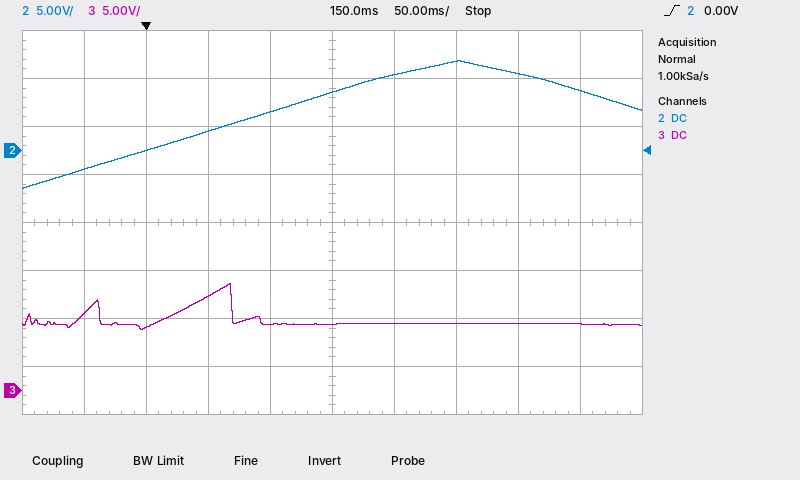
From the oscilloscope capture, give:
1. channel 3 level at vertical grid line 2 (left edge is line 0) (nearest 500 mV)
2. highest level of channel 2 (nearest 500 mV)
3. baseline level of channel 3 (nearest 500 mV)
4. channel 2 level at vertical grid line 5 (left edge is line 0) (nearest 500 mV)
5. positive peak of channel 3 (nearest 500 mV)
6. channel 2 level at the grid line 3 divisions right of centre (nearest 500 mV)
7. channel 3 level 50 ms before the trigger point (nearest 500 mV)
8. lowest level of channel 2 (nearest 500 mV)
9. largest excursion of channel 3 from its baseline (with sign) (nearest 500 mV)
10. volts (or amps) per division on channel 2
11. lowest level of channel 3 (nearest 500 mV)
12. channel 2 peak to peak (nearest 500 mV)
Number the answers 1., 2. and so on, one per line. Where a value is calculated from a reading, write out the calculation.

1. 6.5 V
2. 9.5 V
3. 7.0 V
4. 6.0 V
5. 11.0 V
6. 8.0 V
7. 8.0 V
8. -4.0 V
9. 11.0 V − (7.0 V) = +4.0 V
10. 5 V
11. 6.5 V
12. 9.5 V − (-4.0 V) = 13.5 V
